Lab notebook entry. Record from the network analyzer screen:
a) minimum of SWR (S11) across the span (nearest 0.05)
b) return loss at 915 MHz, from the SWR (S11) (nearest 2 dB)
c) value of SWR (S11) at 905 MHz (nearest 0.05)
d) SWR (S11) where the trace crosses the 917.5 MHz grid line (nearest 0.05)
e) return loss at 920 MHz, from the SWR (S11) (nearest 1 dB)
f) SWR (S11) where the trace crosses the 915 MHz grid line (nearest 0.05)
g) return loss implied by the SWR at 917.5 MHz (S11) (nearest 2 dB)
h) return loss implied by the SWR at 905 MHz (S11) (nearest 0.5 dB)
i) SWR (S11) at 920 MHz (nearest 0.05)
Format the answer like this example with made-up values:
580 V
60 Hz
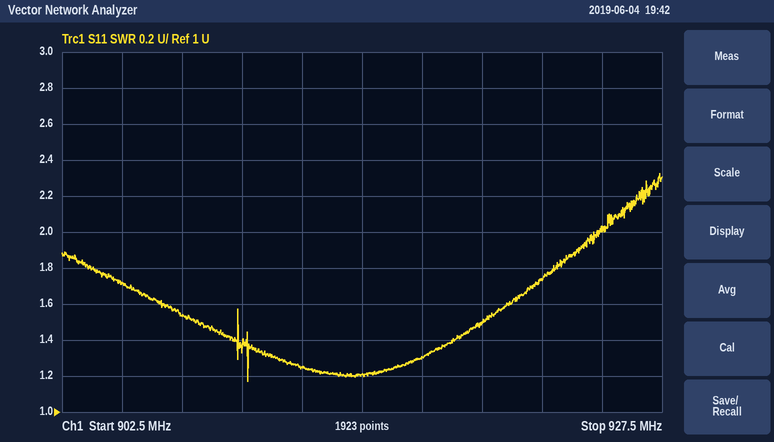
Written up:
1.15
20 dB
1.70
1.30
14 dB
1.20
18 dB
11.5 dB
1.50
